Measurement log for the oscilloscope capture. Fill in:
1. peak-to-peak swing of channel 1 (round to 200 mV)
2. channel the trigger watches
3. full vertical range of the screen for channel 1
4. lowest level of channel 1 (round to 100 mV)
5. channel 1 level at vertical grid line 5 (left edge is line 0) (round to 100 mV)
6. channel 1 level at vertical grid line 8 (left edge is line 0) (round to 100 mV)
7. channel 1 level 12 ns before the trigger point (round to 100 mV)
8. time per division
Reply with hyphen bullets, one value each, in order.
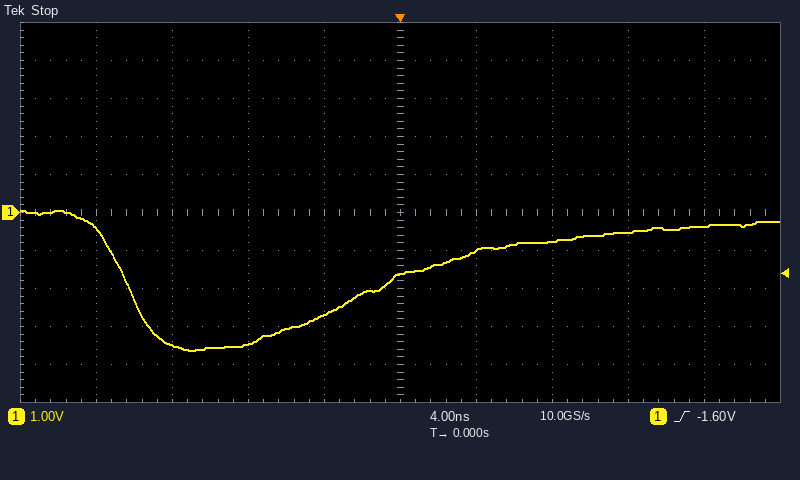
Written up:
- 3.6 V
- channel 1
- 10 V
- -3.6 V
- -1.6 V
- -500 mV
- -3.5 V
- 4 ns
